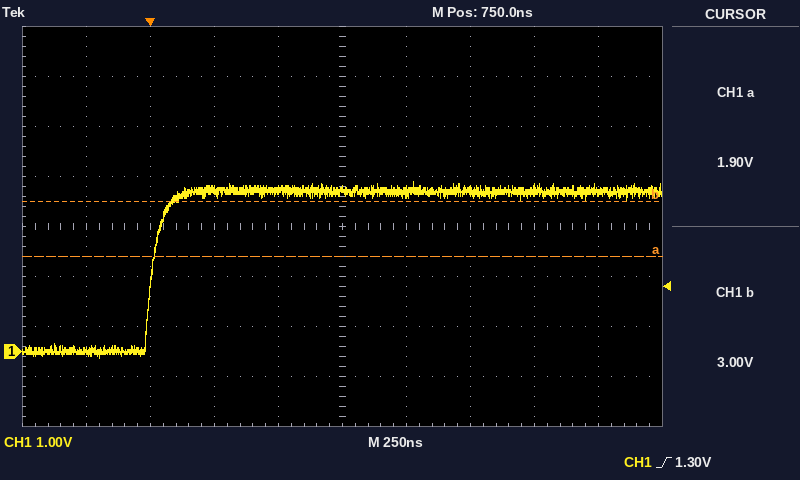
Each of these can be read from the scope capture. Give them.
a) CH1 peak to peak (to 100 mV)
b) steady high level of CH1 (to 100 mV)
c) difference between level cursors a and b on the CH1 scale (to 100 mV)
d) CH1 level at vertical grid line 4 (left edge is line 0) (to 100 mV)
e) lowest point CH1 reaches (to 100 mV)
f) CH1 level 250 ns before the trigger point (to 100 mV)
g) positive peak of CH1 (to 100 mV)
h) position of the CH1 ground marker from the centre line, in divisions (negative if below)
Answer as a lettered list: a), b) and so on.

a) 3.5 V
b) 3.2 V
c) 1.1 V
d) 3.2 V
e) -100 mV
f) 0.0 V
g) 3.4 V
h) -2.5 div
